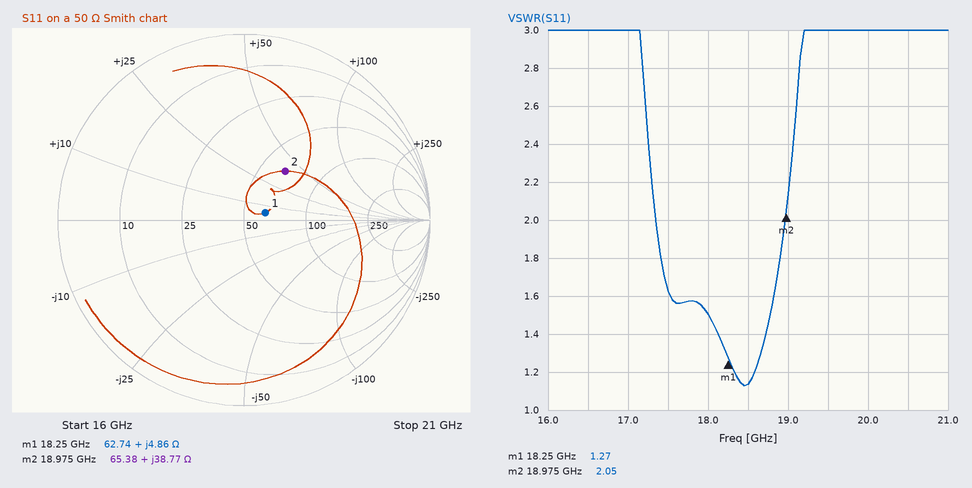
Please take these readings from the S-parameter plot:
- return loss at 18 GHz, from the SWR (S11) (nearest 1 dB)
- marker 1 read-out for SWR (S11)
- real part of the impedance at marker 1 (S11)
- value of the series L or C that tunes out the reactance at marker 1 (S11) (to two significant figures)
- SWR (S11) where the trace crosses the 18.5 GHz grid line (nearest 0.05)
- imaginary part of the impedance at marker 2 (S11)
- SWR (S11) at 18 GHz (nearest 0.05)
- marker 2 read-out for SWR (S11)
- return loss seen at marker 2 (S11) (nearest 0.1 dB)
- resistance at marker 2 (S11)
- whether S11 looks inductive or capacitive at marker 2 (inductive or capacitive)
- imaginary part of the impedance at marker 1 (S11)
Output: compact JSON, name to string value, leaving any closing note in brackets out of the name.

{"return loss at 18 GHz, from the SWR (S11)": "14 dB", "marker 1 read-out for SWR": "1.27", "real part of the impedance at marker 1": "62.74 Ω", "value of the series L or C that tunes out the reactance at marker 1 (S11)": "1.8 pF", "SWR (S11) where the trace crosses the 18.5 GHz grid line": "1.15", "imaginary part of the impedance at marker 2": "+38.77 Ω", "SWR (S11) at 18 GHz": "1.50", "marker 2 read-out for SWR": "2.05", "return loss seen at marker 2 (S11)": "9.3 dB", "resistance at marker 2": "65.38 Ω", "whether S11 looks inductive or capacitive at marker 2": "inductive", "imaginary part of the impedance at marker 1": "+4.86 Ω"}
